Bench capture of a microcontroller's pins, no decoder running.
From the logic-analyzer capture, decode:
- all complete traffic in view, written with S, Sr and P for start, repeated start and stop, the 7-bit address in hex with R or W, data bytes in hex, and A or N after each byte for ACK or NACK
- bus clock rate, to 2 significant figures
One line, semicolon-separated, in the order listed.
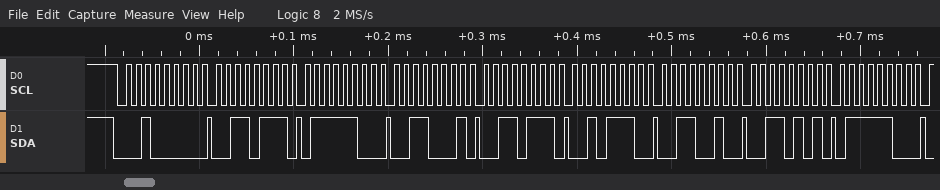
S 10W A 37 A 7C A 31 A 37 A 2E A 32 A 35 A 7C A; 100 kHz
